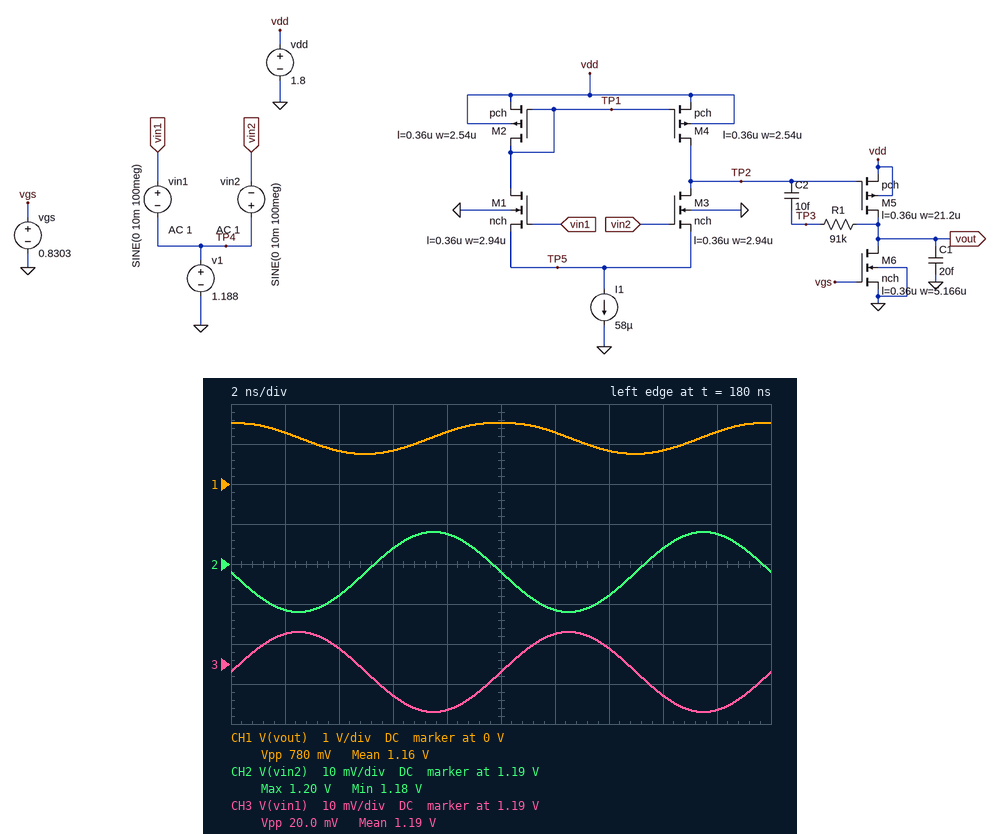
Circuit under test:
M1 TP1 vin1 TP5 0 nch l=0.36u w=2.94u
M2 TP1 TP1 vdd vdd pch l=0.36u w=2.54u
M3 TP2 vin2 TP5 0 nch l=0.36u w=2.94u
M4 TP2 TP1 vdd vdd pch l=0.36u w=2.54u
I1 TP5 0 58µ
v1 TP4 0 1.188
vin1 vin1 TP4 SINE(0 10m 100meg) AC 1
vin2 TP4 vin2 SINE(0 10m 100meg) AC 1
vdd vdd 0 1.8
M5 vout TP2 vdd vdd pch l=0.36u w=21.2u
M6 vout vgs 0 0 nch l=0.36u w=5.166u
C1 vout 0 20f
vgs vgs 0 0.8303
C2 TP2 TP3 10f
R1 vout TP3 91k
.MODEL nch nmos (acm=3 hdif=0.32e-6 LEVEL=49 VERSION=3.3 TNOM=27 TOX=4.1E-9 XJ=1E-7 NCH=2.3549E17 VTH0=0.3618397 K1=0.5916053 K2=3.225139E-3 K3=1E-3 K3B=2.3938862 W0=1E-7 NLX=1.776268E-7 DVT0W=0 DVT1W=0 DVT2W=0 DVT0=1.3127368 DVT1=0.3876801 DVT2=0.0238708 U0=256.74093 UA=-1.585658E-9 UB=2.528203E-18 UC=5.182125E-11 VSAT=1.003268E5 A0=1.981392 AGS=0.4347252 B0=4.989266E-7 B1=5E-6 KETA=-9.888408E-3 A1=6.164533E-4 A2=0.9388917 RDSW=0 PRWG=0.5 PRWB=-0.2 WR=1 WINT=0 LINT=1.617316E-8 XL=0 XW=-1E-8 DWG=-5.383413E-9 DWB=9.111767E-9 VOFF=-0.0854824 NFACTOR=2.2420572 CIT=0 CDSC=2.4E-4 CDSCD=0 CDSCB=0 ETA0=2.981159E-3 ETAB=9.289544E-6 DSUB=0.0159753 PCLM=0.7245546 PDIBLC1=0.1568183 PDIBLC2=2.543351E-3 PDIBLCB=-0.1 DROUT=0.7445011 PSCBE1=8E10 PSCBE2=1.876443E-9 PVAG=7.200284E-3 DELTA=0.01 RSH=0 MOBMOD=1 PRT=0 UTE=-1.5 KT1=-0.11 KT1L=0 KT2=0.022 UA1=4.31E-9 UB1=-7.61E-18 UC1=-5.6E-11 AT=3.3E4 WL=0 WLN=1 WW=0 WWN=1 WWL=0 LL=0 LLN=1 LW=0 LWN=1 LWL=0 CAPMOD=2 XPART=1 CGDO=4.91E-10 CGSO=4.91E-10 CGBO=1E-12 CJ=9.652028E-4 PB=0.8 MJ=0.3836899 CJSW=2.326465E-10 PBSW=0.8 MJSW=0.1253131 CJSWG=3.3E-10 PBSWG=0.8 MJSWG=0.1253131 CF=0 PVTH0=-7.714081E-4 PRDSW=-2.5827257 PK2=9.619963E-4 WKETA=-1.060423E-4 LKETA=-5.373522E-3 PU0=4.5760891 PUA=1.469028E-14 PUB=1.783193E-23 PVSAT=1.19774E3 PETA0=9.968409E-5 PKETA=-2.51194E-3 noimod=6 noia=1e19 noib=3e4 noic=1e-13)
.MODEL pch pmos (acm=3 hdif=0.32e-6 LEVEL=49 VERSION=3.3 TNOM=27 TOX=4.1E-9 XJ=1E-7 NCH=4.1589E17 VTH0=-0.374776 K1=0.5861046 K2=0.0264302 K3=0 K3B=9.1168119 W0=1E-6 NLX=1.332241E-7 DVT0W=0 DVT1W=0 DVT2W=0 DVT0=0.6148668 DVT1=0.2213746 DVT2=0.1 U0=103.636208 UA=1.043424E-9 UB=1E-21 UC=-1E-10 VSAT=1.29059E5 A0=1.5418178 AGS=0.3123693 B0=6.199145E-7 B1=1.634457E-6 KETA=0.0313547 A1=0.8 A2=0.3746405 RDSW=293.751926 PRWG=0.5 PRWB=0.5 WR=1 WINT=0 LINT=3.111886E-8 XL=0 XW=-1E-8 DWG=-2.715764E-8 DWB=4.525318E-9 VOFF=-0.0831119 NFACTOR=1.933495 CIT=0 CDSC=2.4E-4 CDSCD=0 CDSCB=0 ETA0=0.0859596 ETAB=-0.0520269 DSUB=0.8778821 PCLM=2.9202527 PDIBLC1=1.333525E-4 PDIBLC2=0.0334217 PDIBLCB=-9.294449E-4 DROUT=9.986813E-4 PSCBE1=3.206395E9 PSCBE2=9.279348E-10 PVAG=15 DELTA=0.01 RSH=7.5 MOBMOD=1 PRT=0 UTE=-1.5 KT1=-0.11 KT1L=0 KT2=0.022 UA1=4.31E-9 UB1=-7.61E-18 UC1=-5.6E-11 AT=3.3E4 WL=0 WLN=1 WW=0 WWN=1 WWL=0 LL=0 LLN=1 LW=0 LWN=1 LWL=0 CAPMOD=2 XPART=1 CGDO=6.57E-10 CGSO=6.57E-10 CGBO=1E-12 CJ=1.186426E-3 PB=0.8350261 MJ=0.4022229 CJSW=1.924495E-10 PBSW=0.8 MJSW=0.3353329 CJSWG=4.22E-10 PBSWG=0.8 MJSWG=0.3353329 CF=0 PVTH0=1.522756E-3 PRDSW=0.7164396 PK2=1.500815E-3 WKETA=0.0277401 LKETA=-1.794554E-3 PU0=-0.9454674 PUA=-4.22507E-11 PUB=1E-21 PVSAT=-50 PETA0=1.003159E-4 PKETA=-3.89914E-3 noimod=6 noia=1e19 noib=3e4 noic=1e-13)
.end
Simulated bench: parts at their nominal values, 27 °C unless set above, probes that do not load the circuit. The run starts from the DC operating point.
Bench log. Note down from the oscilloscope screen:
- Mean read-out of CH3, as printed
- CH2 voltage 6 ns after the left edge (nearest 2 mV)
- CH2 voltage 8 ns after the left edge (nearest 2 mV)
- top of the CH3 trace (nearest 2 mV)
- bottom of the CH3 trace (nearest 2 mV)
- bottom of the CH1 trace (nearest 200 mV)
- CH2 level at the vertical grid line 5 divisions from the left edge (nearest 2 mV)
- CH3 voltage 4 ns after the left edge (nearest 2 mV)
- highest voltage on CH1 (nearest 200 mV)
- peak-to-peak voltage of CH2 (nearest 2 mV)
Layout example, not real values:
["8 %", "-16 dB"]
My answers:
["1.19 V", "1.194 V", "1.198 V", "1.198 V", "1.178 V", "800 mV", "1.188 V", "1.194 V", "1.6 V", "20 mV"]
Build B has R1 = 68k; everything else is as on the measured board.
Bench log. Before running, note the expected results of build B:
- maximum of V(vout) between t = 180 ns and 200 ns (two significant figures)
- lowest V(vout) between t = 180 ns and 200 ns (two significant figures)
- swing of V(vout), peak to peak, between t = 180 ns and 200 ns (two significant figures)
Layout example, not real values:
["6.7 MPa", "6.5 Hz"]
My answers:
["1.5 V", "770 mV", "760 mV"]
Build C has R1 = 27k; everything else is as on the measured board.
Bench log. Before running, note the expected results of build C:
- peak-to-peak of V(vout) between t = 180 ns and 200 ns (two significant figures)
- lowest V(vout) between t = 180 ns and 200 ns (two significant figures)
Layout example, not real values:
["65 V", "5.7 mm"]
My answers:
["730 mV", "790 mV"]
